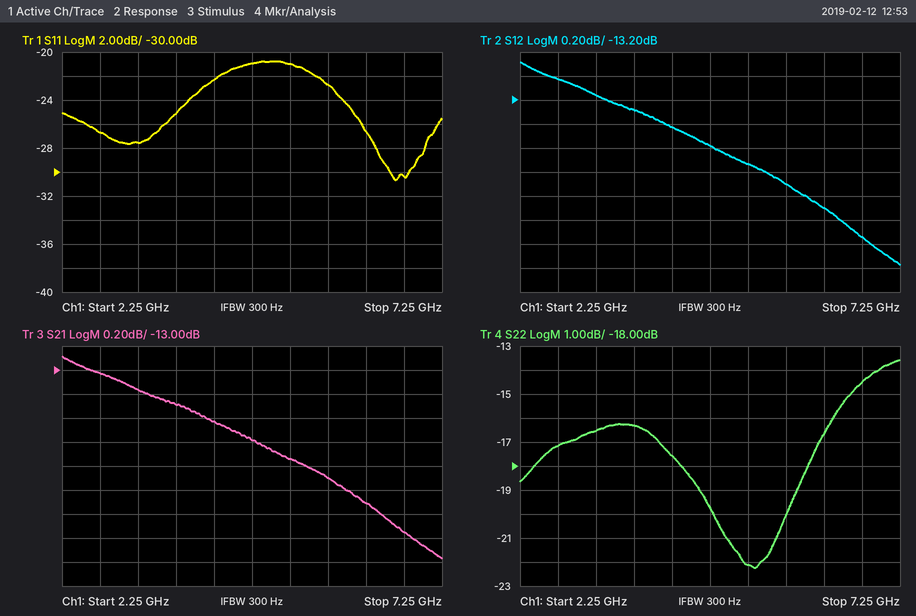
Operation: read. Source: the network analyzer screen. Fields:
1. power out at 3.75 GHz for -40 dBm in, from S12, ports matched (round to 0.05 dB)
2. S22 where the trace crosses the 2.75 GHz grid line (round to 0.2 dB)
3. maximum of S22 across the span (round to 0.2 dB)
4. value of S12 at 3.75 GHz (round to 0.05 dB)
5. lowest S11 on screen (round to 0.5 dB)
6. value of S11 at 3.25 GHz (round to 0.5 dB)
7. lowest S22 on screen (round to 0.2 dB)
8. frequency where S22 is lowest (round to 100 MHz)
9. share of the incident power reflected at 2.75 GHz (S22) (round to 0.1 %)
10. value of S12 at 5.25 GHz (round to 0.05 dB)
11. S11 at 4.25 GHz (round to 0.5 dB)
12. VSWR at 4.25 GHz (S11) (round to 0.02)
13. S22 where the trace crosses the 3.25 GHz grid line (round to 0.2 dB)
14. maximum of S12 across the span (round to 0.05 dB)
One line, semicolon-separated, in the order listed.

-53.30 dBm; -17.2 dB; -13.6 dB; -13.30 dB; -30.5 dB; -27.5 dB; -22.2 dB; 5.3 GHz; 1.9 %; -13.75 dB; -22.5 dB; 1.16; -16.6 dB; -12.90 dB
